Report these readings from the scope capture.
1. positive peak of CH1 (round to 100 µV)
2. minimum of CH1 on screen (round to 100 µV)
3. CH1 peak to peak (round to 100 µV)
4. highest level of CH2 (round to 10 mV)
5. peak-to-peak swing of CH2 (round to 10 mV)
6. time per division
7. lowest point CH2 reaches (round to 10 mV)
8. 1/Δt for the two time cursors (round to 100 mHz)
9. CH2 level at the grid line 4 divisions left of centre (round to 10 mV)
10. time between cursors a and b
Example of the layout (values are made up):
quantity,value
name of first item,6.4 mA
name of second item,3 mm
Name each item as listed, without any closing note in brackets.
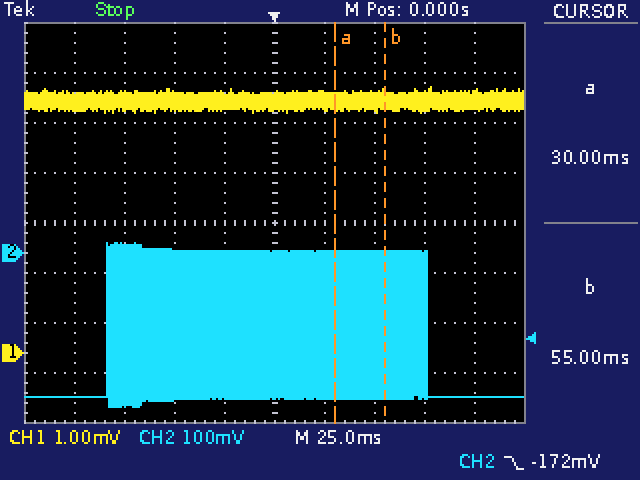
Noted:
quantity,value
positive peak of CH1,5.3 mV
minimum of CH1 on screen,4.8 mV
CH1 peak to peak,500 µV
highest level of CH2,20 mV
peak-to-peak swing of CH2,330 mV
time per division,25 ms
lowest point CH2 reaches,-310 mV
1/Δt for the two time cursors,40.0 Hz
CH2 level at the grid line 4 divisions left of centre,-290 mV
time between cursors a and b,25.0 ms
